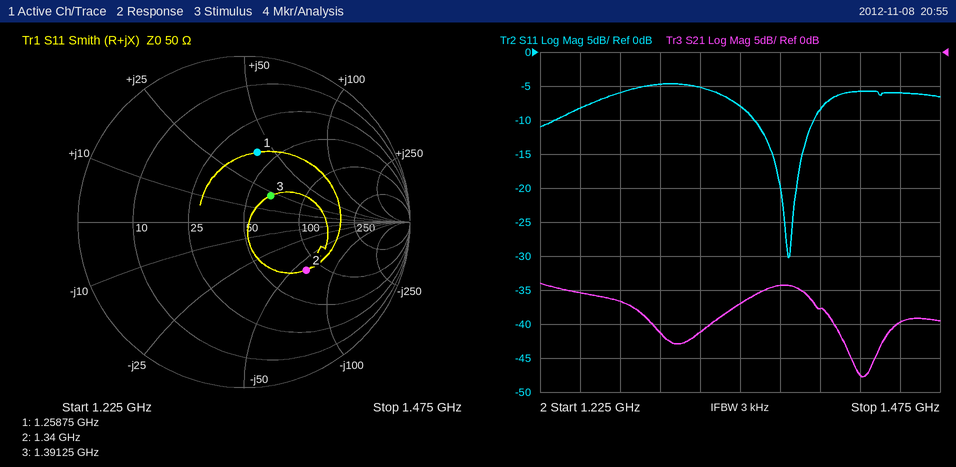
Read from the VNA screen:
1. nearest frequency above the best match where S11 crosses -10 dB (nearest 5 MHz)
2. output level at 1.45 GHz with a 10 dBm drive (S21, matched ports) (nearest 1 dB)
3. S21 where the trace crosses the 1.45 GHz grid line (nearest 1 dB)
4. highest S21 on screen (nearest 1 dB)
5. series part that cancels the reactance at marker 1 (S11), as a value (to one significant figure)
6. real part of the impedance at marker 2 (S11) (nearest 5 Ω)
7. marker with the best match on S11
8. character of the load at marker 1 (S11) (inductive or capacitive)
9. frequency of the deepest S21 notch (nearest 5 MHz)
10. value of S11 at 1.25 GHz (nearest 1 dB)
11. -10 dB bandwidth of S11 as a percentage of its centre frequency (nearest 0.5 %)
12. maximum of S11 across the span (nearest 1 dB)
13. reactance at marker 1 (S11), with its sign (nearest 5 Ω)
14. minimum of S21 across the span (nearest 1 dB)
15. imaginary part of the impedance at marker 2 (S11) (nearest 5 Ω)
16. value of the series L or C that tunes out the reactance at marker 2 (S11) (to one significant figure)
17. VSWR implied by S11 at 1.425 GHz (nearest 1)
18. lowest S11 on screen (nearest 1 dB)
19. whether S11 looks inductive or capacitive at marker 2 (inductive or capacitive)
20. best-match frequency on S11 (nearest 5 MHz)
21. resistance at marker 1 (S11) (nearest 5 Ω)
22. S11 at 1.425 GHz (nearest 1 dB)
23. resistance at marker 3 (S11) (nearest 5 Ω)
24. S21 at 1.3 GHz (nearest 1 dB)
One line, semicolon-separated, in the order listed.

1.395 GHz; -30 dBm; -40 dB; -34 dB; 3 pF; 80 Ω; marker 3; inductive; 1.425 GHz; -8 dB; 2.5 %; -5 dB; +40 Ω; -48 dB; -60 Ω; 7 nH; 3; -30 dB; capacitive; 1.380 GHz; 40 Ω; -6 dB; 65 Ω; -41 dB
